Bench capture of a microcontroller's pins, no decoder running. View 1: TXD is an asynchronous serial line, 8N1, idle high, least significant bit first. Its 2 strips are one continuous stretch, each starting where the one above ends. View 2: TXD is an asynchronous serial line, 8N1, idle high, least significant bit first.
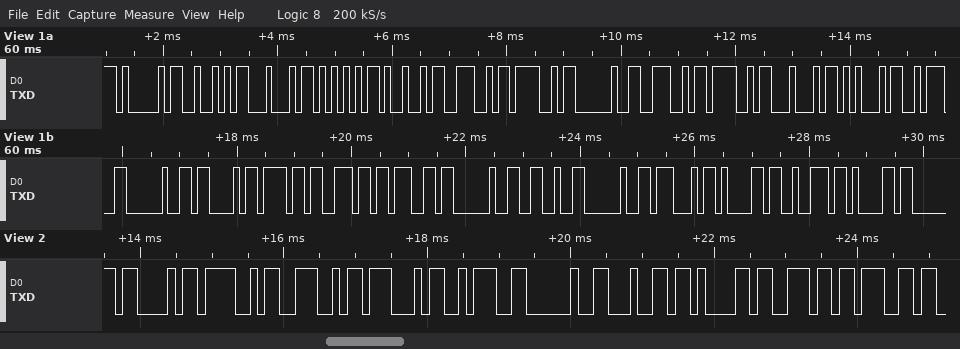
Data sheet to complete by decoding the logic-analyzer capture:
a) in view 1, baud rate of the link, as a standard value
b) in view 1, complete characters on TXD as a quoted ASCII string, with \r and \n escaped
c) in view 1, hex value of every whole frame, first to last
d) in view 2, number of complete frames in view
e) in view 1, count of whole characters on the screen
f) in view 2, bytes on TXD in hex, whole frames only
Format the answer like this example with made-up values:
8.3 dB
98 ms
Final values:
9600 baud
"ARDUINO NODE: Cong & Gara"
41 52 44 55 49 4E 4F 20 4E 4F 44 45 3A 20 43 6F 6E 67 20 26 20 47 61 72 61
10
25
43 4F 4E 47 3A 20 64 61 6E 67
